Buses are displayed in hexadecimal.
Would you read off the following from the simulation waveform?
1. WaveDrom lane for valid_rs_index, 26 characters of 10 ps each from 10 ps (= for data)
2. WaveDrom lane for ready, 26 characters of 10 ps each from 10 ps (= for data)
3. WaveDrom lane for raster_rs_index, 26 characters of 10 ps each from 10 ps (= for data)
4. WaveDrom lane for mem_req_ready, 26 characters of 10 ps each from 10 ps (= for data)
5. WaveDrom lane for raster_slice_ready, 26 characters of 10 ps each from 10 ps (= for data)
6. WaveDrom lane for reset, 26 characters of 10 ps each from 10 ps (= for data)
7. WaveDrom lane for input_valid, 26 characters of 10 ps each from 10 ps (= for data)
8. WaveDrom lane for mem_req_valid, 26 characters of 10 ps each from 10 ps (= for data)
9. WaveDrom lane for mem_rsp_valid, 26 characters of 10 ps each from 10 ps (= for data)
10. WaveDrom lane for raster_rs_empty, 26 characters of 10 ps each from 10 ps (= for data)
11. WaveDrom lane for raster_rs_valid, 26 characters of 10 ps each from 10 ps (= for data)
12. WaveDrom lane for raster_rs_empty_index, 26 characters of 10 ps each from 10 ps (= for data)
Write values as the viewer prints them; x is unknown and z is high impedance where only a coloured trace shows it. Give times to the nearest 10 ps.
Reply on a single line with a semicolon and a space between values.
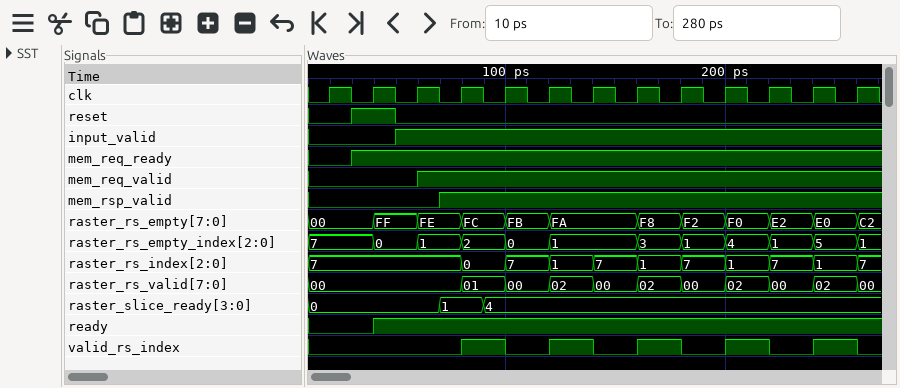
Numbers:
{name: 'valid_rs_index', wave: '0......1.0.1.0.1.0.1.0.1.0'}; {name: 'ready', wave: '0..1......................'}; {name: 'raster_rs_index', wave: '=......=.=.=.=.=.=.=.=.=.=', data: '7 0 7 1 7 1 7 1 7 1 7'}; {name: 'mem_req_ready', wave: '0.1.......................'}; {name: 'raster_slice_ready', wave: '=.....=.=.................', data: '0 1 4'}; {name: 'reset', wave: '0.1.0.....................'}; {name: 'input_valid', wave: '0...1.....................'}; {name: 'mem_req_valid', wave: '0....1....................'}; {name: 'mem_rsp_valid', wave: '0.....1...................'}; {name: 'raster_rs_empty', wave: '=..=.=.=.=.=...=.=.=.=.=.=', data: '00 FF FE FC FB FA F8 F2 F0 E2 E0 C2'}; {name: 'raster_rs_valid', wave: '=......=.=.=.=.=.=.=.=.=.=', data: '00 01 00 02 00 02 00 02 00 02 00'}; {name: 'raster_rs_empty_index', wave: '=..=.=.=.=.=...=.=.=.=.=.=', data: '7 0 1 2 0 1 3 1 4 1 5 1'}
